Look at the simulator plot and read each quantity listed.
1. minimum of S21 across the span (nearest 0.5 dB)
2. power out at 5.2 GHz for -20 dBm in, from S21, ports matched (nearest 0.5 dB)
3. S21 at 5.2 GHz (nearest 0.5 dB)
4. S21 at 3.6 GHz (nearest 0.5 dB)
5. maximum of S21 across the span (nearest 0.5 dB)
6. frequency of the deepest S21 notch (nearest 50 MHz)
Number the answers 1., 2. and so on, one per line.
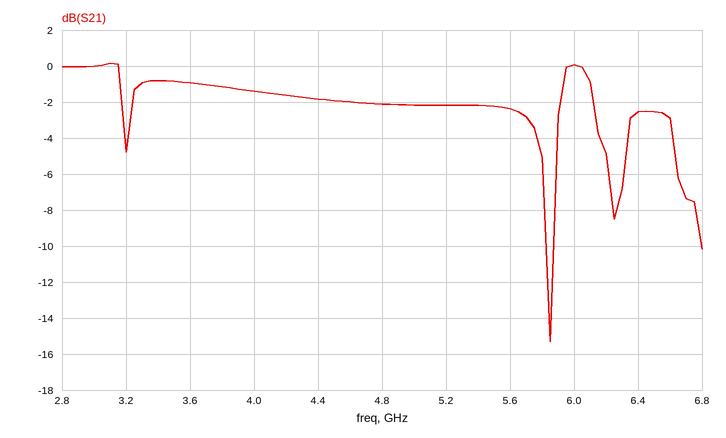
1. -15.5 dB
2. -22.0 dBm
3. -2.0 dB
4. -1.0 dB
5. 0.0 dB
6. 5.85 GHz
